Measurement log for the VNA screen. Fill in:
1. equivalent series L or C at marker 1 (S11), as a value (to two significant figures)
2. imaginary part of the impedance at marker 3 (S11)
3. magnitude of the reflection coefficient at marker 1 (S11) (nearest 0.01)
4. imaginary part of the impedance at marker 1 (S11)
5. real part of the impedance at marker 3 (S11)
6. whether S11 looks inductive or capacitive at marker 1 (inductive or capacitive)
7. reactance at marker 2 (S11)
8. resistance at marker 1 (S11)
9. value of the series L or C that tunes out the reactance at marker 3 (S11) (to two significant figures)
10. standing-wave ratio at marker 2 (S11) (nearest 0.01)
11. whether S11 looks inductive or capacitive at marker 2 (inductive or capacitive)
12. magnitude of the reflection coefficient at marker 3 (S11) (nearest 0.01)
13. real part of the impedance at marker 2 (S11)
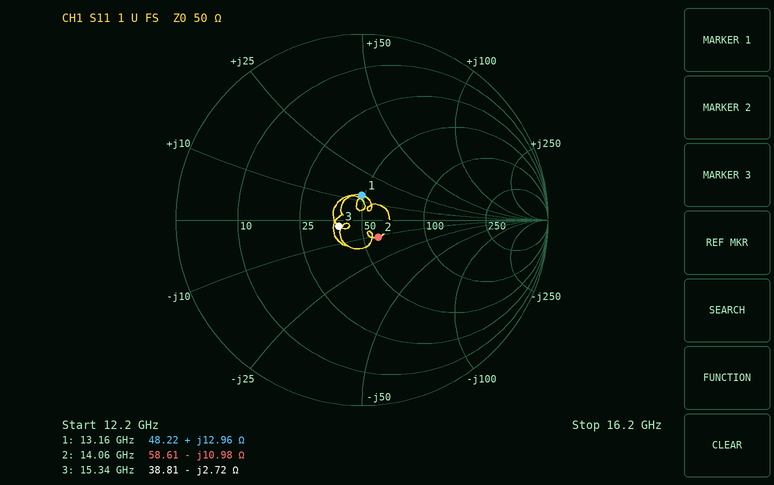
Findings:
160 pH
-2.72 Ω
0.13
+12.96 Ω
38.81 Ω
inductive
-10.98 Ω
48.22 Ω
28 pH
1.29
capacitive
0.13
58.61 Ω
